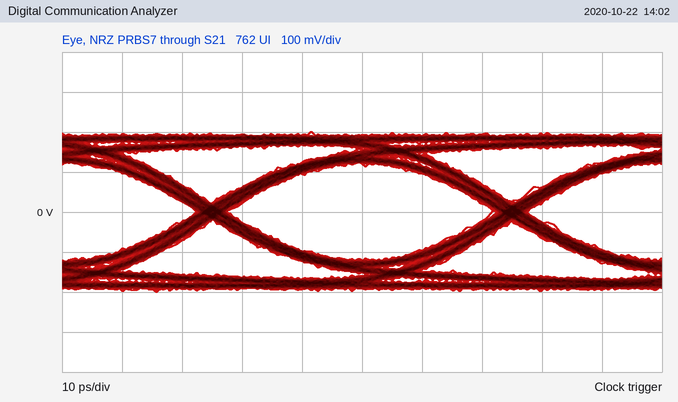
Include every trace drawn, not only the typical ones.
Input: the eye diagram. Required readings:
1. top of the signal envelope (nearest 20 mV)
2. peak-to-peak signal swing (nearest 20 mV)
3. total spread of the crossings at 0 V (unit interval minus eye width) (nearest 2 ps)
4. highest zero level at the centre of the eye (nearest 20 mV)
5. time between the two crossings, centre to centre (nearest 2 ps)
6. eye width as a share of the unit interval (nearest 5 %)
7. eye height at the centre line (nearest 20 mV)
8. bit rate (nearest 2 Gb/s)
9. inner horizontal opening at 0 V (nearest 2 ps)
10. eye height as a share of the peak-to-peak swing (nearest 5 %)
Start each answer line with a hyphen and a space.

- 200 mV
- 400 mV
- 6 ps
- -120 mV
- 50 ps
- 90 %
- 240 mV
- 20 Gb/s
- 44 ps
- 60 %
